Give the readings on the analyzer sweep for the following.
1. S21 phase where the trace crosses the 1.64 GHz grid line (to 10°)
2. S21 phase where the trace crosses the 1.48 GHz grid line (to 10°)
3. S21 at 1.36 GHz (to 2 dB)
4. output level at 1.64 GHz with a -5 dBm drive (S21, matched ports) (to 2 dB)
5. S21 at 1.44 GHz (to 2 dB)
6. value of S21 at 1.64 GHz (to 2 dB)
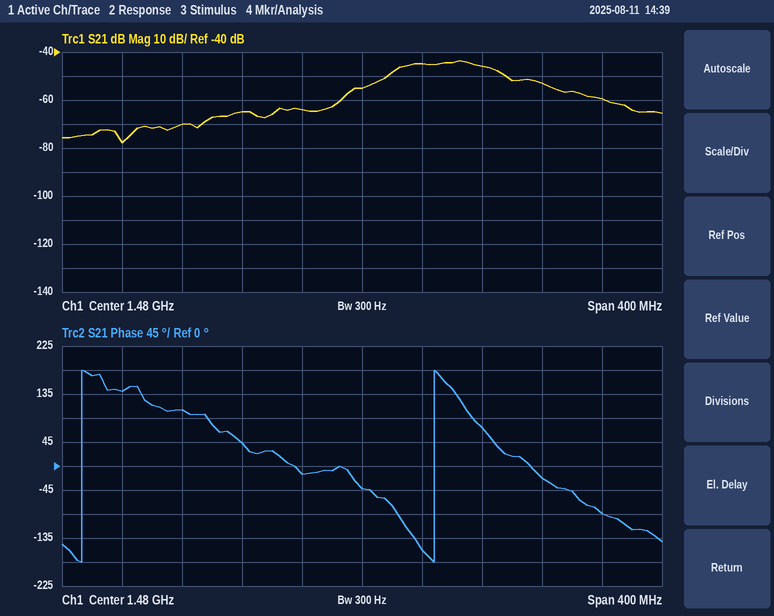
-90°
-40°
-70 dB
-64 dBm
-64 dB
-60 dB
